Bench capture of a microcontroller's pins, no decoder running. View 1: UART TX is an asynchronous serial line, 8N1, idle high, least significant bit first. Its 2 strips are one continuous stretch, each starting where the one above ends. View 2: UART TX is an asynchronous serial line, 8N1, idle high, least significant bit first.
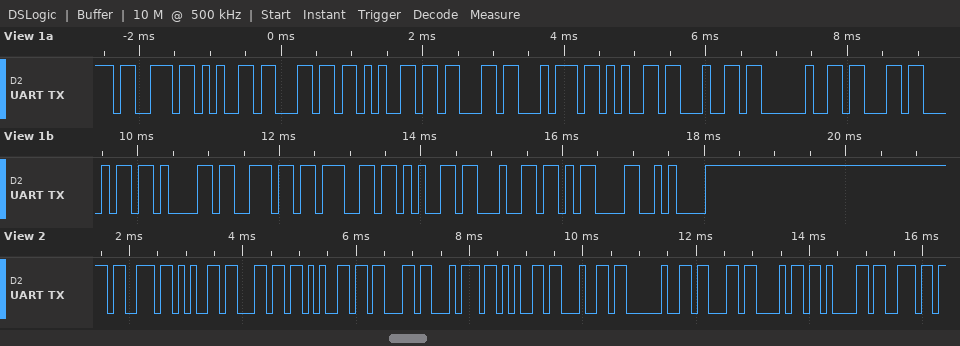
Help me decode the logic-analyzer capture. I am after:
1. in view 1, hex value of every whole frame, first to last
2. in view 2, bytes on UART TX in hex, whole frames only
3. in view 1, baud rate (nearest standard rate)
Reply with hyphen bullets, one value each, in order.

- 73 65 6C 65 63 74 65 64 20 63 68 61 6E 67 65 64 0D 0A
- 0x73 0x65 0x6C 0x65 0x63 0x74 0x65 0x64 0x20 0x63 0x68 0x61 0x6E
- 9600 baud
